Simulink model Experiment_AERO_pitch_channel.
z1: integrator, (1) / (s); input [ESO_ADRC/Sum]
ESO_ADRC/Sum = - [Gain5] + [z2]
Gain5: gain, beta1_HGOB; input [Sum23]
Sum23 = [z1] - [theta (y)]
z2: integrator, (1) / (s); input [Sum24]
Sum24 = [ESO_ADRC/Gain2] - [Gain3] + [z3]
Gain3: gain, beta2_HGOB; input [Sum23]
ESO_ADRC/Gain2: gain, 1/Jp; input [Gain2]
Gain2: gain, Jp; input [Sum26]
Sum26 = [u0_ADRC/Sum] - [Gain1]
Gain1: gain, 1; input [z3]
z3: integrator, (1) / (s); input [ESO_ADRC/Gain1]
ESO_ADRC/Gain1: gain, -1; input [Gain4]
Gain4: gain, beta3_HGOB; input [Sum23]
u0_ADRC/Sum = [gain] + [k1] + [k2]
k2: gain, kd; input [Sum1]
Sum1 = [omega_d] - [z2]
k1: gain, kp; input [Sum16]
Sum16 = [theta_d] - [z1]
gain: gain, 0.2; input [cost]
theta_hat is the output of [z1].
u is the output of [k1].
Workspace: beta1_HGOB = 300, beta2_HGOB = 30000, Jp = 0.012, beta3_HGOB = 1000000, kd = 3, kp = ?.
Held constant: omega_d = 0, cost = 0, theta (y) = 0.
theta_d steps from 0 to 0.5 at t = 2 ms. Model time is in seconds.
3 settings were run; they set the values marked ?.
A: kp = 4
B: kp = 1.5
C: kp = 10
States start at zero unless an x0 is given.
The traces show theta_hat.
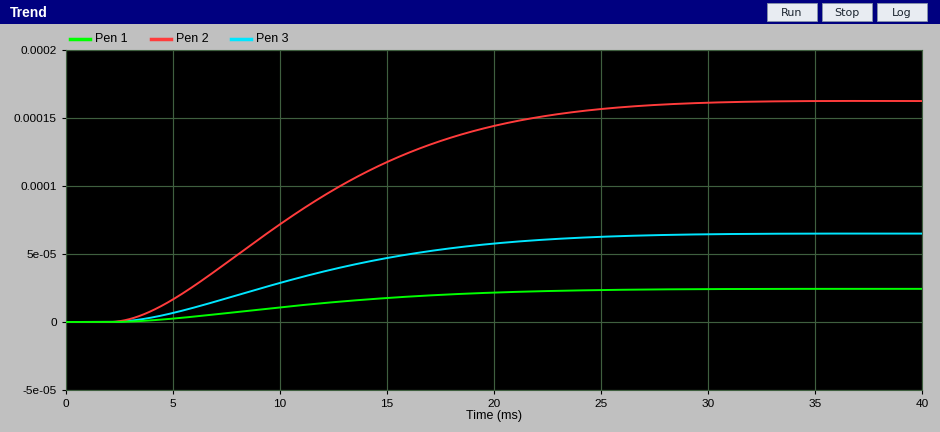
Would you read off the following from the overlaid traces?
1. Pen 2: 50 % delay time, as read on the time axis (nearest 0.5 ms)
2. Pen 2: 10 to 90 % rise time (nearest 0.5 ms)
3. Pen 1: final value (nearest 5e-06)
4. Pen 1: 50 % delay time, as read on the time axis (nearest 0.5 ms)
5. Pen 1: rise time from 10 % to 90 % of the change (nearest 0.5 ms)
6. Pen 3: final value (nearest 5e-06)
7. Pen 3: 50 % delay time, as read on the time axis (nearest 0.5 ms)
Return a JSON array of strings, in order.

["11.0 ms", "15.5 ms", "0.000025", "11.0 ms", "15.5 ms", "0.000065", "11.0 ms"]
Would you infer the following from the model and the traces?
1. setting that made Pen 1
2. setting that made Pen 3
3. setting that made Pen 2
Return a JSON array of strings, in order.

["B", "A", "C"]
